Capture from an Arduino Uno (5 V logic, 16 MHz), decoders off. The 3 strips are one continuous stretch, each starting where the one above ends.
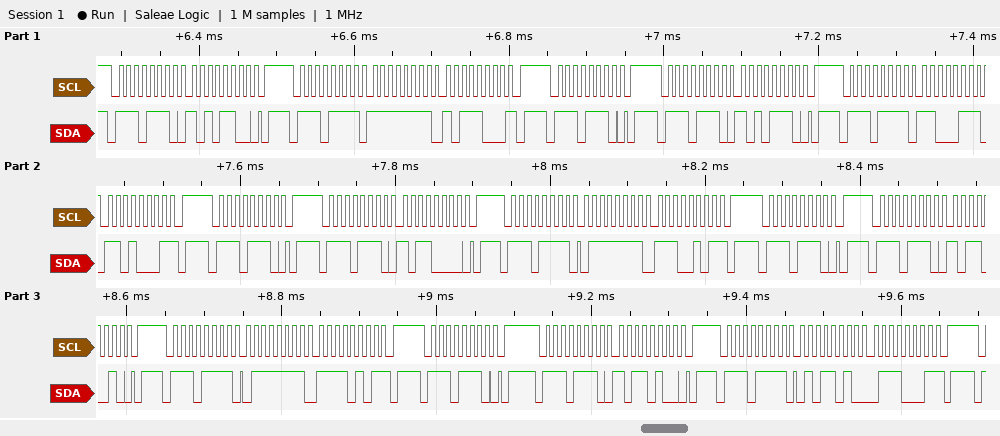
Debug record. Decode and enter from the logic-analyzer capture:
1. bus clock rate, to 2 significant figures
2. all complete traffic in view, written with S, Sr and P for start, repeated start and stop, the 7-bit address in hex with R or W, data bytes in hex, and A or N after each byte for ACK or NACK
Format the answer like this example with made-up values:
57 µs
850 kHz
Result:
100 kHz
S 77W A AC A P S 77R A FF A B8 N P S 77W A P S 77W A AE A P S 77R A C7 A D1 N P S 77W A P S 77W A B0 A P S 77R A 7F A E5 N P S 77W A P S 77W A B2 A P S 77R A 7F A F5 N P S 77W A P S 77W A B4 A P S 77R A 5A A 71 N P
